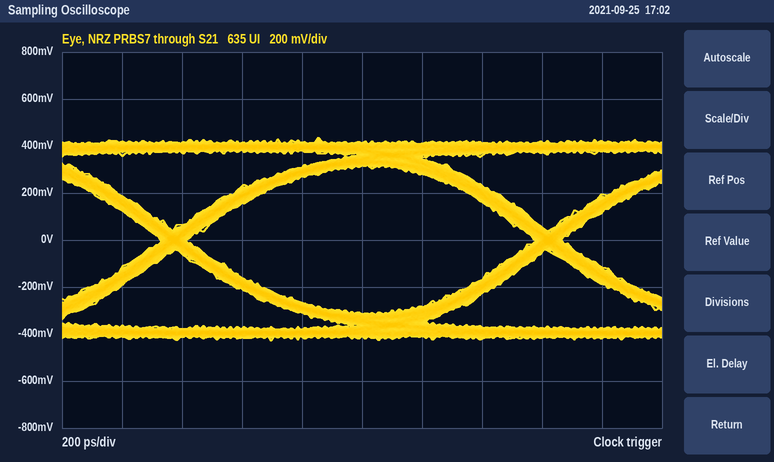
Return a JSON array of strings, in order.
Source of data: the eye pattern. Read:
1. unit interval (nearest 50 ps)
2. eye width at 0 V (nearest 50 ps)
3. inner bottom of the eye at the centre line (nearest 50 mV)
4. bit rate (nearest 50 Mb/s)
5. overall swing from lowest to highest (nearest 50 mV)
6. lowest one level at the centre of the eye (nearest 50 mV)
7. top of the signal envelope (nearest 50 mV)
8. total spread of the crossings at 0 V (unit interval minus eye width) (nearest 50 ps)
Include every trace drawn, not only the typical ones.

["1.25 ns", "1.15 ns", "-300 mV", "800 Mb/s", "850 mV", "300 mV", "450 mV", "100 ps"]
